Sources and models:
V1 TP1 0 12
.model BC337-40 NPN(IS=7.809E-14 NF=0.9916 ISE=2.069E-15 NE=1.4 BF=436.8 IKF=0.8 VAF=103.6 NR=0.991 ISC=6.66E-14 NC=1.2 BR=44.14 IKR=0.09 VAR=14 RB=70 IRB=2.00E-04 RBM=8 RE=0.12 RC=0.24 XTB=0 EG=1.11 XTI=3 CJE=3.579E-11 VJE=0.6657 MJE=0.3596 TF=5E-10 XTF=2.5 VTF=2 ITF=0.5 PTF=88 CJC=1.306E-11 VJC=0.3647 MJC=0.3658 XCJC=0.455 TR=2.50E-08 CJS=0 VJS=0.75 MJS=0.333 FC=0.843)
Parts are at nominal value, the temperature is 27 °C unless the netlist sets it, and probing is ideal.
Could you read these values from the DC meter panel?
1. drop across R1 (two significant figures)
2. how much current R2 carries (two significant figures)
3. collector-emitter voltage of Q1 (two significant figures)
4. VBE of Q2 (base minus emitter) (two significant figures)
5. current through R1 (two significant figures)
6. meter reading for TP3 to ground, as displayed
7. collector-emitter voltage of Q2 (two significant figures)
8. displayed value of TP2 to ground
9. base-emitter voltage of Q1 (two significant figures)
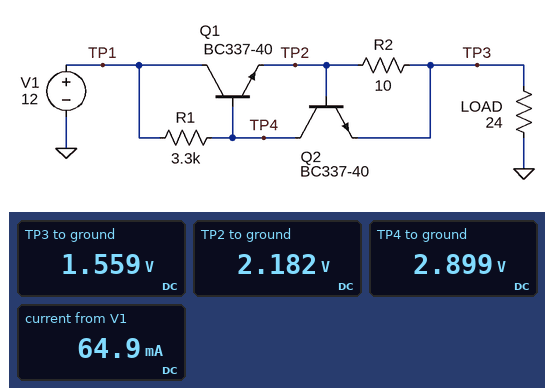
9.1 V
62 mA
9.8 V
620 mV
2.8 mA
1.559 V
1.3 V
2.182 V
720 mV
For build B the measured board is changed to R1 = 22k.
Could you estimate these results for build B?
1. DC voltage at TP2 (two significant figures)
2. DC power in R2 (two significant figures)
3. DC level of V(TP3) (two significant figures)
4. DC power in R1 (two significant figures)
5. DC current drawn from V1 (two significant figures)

1.9 V
32 mW
1.4 V
4.0 mW
57 mA
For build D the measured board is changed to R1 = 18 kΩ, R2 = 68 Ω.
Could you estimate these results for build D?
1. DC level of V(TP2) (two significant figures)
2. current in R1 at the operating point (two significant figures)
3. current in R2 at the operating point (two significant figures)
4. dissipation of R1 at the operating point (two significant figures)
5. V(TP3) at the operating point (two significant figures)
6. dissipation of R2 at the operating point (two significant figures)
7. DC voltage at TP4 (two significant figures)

800 mV
590 µA
8.6 mA
6.2 mW
220 mV
5.0 mW
1.5 V
